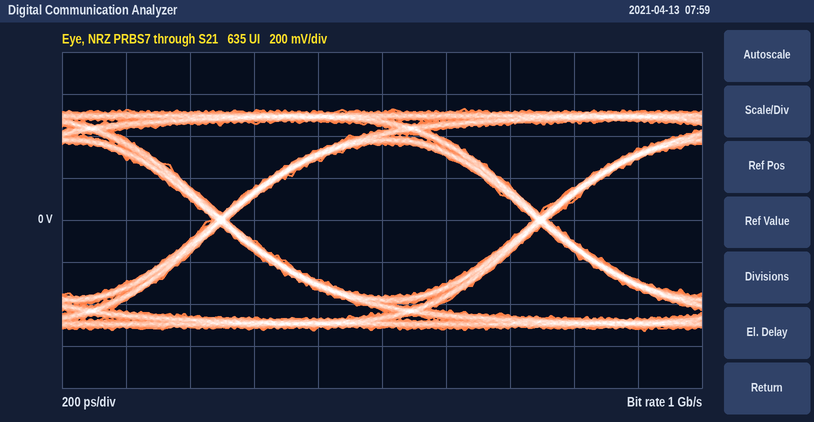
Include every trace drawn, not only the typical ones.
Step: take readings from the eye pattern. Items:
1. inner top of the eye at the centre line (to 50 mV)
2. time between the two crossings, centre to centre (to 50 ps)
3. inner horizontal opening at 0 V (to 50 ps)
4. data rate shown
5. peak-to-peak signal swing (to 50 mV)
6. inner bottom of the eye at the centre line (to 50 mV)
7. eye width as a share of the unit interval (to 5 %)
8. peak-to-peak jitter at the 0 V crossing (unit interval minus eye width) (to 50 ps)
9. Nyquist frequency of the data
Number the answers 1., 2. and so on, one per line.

1. 350 mV
2. 1.00 ns
3. 950 ps
4. 1 Gb/s
5. 1.05 V
6. -350 mV
7. 95 %
8. 50 ps
9. 500 MHz
